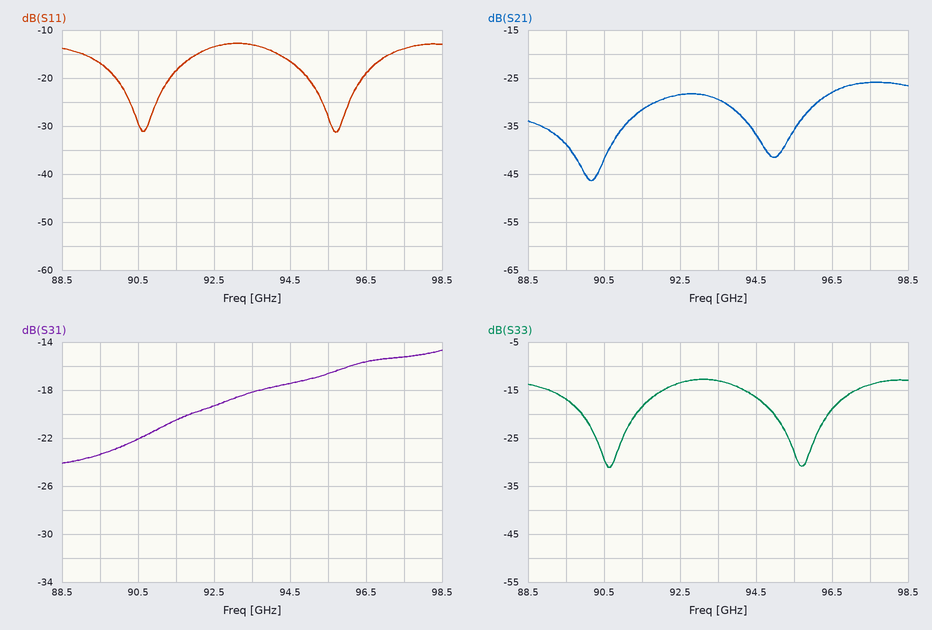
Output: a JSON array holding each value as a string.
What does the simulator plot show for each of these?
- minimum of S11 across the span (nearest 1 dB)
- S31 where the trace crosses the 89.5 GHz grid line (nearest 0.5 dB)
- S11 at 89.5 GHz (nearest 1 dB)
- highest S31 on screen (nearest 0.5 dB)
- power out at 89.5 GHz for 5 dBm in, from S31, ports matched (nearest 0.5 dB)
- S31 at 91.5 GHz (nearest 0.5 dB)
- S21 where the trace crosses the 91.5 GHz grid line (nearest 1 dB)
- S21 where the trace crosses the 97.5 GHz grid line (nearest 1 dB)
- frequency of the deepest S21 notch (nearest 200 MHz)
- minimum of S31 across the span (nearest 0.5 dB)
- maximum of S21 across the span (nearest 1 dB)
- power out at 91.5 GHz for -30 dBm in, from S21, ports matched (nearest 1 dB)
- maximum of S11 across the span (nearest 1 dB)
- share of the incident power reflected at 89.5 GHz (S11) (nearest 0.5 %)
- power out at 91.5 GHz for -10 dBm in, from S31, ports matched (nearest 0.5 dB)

["-31 dB", "-23.5 dB", "-17 dB", "-14.5 dB", "-18.5 dBm", "-20.5 dB", "-32 dB", "-26 dB", "90.2 GHz", "-24.0 dB", "-26 dB", "-62 dBm", "-13 dB", "2.0 %", "-30.5 dBm"]
